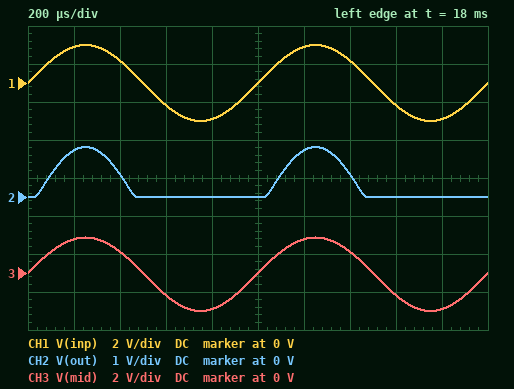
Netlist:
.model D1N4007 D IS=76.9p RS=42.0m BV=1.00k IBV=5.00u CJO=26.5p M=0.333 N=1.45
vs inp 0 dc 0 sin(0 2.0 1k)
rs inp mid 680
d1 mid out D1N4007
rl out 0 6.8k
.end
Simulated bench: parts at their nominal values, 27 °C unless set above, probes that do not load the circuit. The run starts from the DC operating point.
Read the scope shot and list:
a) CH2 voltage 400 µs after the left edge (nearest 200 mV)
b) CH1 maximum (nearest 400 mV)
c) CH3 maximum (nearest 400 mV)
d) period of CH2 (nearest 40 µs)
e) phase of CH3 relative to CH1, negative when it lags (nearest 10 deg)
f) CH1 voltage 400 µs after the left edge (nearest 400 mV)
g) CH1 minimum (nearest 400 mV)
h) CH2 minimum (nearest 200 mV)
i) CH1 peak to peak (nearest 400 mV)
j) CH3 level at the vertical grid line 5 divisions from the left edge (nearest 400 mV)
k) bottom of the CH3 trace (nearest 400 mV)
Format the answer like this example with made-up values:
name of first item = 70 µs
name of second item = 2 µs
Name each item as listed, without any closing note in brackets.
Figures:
CH2 voltage 400 µs after the left edge = 600 mV
CH1 maximum = 2.0 V
CH3 maximum = 2.0 V
period of CH2 = 1.00 ms
phase of CH3 relative to CH1, negative when it lags = 0 deg
CH1 voltage 400 µs after the left edge = 1.2 V
CH1 minimum = -2.0 V
CH2 minimum = 0 V
CH1 peak to peak = 4.0 V
CH3 level at the vertical grid line 5 divisions from the left edge = 0 V
bottom of the CH3 trace = -2.0 V
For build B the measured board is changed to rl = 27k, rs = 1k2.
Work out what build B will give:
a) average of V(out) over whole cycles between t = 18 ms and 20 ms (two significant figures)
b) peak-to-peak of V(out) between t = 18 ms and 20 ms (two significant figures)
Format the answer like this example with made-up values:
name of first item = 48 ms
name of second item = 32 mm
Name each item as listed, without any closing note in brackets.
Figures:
average of V(out) over whole cycles between t = 18 ms and 20 ms = 400 mV
peak-to-peak of V(out) between t = 18 ms and 20 ms = 1.4 V
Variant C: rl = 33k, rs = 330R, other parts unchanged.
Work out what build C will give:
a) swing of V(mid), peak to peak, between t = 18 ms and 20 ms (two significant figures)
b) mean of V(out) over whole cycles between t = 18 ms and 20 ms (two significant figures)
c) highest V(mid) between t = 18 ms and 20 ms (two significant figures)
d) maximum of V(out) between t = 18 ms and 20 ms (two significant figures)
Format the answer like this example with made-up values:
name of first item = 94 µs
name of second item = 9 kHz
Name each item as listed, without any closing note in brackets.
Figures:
swing of V(mid), peak to peak, between t = 18 ms and 20 ms = 4.0 V
mean of V(out) over whole cycles between t = 18 ms and 20 ms = 410 mV
highest V(mid) between t = 18 ms and 20 ms = 2.0 V
maximum of V(out) between t = 18 ms and 20 ms = 1.5 V
